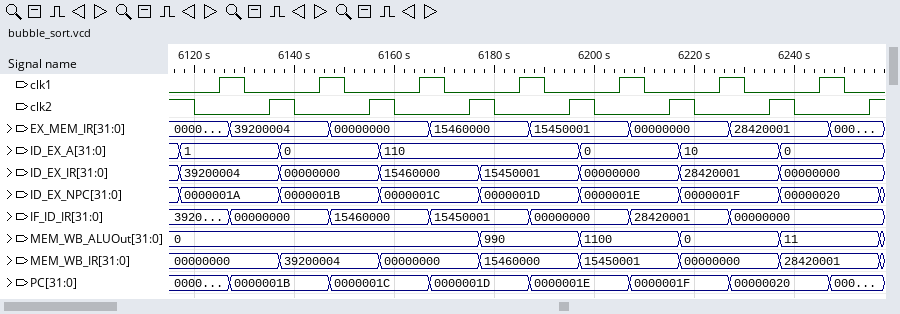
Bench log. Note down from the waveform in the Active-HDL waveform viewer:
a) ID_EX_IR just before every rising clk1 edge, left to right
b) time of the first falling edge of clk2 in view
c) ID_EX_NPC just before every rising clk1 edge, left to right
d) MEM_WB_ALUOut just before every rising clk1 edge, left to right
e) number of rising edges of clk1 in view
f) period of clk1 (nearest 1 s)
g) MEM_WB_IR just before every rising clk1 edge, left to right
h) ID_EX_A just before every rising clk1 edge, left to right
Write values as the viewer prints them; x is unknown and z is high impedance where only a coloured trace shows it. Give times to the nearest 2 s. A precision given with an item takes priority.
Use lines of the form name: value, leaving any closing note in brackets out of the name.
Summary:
ID_EX_IR just before every rising clk1 edge, left to right: 39200004, 00000000, 15460000, 15450001, 00000000, 28420001, 00000000
time of the first falling edge of clk2 in view: 6120 s
ID_EX_NPC just before every rising clk1 edge, left to right: 0000001A, 0000001B, 0000001C, 0000001D, 0000001E, 0000001F, 00000020
MEM_WB_ALUOut just before every rising clk1 edge, left to right: 0, 0, 0, 990, 1100, 0, 11
number of rising edges of clk1 in view: 7
period of clk1: 20 s
MEM_WB_IR just before every rising clk1 edge, left to right: 00000000, 39200004, 00000000, 15460000, 15450001, 00000000, 28420001
ID_EX_A just before every rising clk1 edge, left to right: 1, 0, 110, 110, 0, 10, 0
